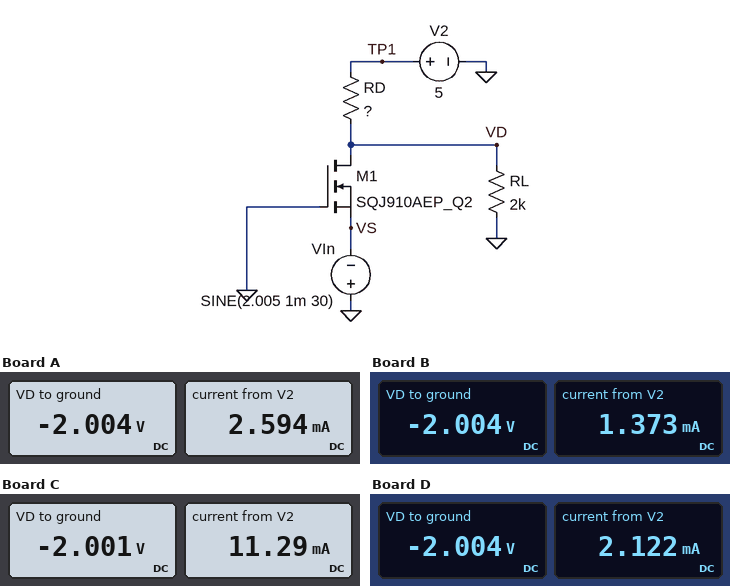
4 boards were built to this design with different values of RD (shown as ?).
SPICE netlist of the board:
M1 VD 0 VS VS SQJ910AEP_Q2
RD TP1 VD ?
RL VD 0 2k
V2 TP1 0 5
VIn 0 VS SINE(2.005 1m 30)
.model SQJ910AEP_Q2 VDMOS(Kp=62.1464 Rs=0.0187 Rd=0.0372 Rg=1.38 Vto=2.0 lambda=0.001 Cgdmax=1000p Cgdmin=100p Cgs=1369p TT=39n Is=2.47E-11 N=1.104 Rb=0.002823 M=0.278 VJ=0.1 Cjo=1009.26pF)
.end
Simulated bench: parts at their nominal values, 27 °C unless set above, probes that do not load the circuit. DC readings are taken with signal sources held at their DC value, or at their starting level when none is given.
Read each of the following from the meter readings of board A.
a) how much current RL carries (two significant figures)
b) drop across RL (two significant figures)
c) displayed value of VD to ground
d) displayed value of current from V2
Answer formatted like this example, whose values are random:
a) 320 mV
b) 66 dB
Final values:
a) 1.0 mA
b) 2.0 V
c) -2.004 V
d) 2.594 mA
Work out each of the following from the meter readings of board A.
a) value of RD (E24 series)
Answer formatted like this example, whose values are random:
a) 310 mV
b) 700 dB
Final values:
a) 2.7 kΩ
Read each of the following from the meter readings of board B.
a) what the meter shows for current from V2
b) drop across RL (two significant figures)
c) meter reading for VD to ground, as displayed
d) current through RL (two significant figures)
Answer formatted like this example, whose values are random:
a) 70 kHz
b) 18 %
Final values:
a) 1.373 mA
b) 2.0 V
c) -2.004 V
d) 1.0 mA
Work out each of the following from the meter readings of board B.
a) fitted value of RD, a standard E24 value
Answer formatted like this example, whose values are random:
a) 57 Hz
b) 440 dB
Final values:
a) 5.1 kΩ
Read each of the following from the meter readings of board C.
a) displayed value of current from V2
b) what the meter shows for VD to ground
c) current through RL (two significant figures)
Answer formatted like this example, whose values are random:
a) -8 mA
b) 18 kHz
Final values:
a) 11.29 mA
b) -2.001 V
c) 1.0 mA
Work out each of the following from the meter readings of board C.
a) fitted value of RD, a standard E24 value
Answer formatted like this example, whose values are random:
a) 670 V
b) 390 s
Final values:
a) 620 Ω
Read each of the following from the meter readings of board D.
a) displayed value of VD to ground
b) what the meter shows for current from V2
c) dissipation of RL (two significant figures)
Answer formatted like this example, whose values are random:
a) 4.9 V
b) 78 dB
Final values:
a) -2.004 V
b) 2.122 mA
c) 2.0 mW
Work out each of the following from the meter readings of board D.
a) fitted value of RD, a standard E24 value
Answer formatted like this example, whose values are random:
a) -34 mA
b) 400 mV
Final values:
a) 3.3 kΩ
